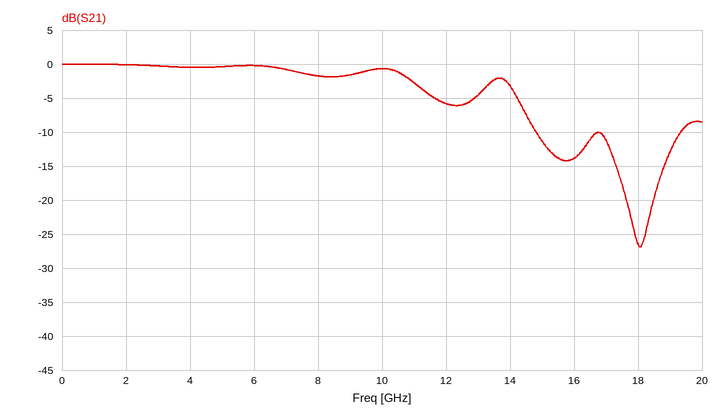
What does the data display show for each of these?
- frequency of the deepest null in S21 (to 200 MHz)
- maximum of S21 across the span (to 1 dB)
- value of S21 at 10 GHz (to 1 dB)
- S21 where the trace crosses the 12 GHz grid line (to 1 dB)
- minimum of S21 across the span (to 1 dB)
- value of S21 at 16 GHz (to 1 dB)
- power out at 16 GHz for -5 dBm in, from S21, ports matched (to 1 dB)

18.0 GHz
0 dB
-1 dB
-6 dB
-27 dB
-14 dB
-19 dBm
